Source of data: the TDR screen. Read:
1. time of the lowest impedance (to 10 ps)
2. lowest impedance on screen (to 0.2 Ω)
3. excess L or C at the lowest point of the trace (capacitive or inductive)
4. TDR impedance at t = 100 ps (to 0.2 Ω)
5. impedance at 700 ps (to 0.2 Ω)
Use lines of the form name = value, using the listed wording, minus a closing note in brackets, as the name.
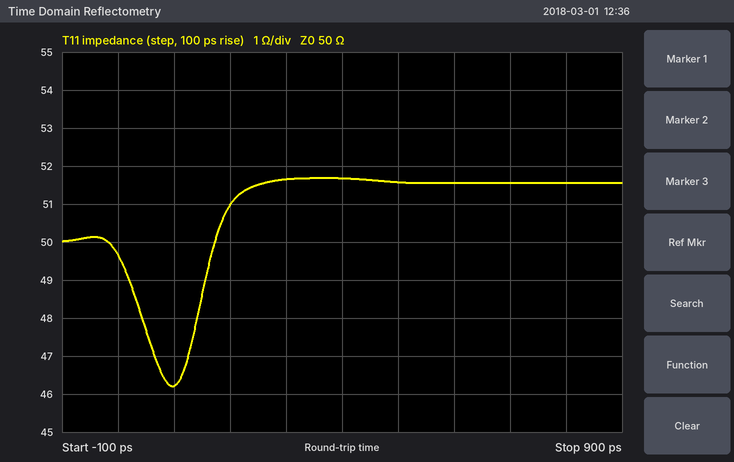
time of the lowest impedance = 100 ps
lowest impedance on screen = 46.2 Ω
excess L or C at the lowest point of the trace = capacitive
TDR impedance at t = 100 ps = 46.2 Ω
impedance at 700 ps = 51.6 Ω
